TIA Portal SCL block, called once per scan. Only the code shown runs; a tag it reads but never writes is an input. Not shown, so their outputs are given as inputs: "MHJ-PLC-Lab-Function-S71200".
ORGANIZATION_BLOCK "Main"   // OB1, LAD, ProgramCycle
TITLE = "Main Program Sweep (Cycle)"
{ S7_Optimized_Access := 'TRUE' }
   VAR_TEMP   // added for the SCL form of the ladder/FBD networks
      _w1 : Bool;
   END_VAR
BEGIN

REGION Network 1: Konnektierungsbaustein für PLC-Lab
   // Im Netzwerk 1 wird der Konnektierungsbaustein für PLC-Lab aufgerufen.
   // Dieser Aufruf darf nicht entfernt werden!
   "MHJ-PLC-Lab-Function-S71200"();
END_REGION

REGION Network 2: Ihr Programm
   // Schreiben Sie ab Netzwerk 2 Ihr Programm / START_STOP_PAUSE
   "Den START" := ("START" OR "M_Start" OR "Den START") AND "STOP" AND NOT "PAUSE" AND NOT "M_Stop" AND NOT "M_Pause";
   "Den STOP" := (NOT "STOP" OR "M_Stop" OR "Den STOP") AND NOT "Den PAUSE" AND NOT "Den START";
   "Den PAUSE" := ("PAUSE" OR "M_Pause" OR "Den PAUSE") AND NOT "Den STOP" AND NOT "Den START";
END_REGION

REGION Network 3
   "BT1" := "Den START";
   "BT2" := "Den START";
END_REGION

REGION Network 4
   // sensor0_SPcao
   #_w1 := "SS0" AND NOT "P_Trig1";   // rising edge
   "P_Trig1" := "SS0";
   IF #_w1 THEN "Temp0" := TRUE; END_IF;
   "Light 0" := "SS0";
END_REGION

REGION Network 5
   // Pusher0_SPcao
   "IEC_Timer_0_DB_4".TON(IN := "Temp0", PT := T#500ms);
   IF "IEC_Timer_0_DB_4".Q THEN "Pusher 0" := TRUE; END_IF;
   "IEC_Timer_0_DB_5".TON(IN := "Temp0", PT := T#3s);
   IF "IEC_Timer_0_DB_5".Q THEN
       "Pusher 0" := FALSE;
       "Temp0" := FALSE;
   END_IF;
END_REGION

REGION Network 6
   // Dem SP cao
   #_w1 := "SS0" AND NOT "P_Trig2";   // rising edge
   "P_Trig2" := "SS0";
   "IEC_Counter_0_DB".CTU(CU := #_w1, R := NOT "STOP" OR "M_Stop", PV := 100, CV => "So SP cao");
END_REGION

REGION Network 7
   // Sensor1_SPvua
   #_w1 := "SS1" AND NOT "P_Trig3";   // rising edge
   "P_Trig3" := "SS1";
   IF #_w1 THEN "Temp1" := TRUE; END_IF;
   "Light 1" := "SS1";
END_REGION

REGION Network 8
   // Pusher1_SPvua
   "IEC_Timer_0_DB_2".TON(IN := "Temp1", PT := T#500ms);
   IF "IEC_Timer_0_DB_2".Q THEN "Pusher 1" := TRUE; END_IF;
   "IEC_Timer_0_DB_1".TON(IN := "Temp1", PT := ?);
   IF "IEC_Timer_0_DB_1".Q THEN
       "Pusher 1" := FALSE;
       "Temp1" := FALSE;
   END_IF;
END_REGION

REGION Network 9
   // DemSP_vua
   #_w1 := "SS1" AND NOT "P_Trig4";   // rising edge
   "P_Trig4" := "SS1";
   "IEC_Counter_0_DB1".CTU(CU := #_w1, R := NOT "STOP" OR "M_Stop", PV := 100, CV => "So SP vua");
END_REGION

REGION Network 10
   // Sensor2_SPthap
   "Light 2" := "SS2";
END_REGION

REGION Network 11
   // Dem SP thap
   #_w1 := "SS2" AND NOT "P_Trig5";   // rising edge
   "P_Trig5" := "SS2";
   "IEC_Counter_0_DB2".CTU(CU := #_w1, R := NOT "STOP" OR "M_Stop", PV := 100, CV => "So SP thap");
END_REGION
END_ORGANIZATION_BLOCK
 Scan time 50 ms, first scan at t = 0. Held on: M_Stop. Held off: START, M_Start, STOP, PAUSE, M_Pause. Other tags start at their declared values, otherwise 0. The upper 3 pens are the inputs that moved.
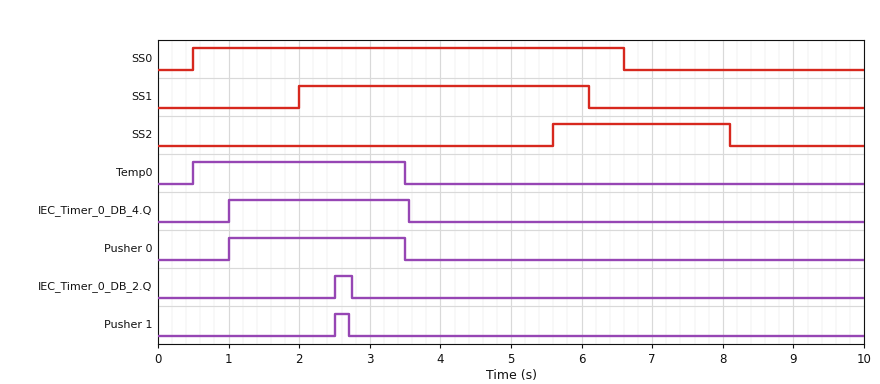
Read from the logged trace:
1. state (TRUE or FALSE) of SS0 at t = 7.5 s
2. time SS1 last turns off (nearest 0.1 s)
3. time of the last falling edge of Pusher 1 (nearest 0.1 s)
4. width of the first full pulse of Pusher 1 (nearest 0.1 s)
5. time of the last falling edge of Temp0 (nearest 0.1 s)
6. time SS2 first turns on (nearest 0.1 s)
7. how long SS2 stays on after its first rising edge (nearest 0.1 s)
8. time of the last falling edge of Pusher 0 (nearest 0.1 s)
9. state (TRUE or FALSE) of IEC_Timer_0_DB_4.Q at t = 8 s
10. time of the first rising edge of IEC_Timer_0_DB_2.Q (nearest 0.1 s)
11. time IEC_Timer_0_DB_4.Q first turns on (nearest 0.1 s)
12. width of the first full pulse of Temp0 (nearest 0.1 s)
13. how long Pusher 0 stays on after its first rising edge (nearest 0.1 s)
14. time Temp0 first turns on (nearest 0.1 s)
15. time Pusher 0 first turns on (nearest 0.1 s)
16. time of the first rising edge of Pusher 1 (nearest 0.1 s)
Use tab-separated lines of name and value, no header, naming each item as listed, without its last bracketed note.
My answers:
state (TRUE or FALSE) of SS0 at t = 7.5 s	FALSE
time SS1 last turns off	6.1 s
time of the last falling edge of Pusher 1	2.7 s
width of the first full pulse of Pusher 1	0.2 s
time of the last falling edge of Temp0	3.5 s
time SS2 first turns on	5.6 s
how long SS2 stays on after its first rising edge	2.5 s
time of the last falling edge of Pusher 0	3.5 s
state (TRUE or FALSE) of IEC_Timer_0_DB_4.Q at t = 8 s	FALSE
time of the first rising edge of IEC_Timer_0_DB_2.Q	2.5 s
time IEC_Timer_0_DB_4.Q first turns on	1.0 s
width of the first full pulse of Temp0	3.0 s
how long Pusher 0 stays on after its first rising edge	2.5 s
time Temp0 first turns on	0.5 s
time Pusher 0 first turns on	1.0 s
time of the first rising edge of Pusher 1	2.5 s
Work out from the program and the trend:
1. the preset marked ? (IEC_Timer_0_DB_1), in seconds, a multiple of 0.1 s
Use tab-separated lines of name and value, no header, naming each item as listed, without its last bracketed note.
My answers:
the preset marked ? (IEC_Timer_0_DB_1), in seconds, a multiple of 0.1 s	0.7 s
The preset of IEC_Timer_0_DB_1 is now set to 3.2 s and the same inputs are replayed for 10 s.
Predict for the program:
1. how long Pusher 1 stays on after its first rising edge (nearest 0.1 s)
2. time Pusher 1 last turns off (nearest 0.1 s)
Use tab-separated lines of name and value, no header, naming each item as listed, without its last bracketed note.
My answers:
how long Pusher 1 stays on after its first rising edge	2.7 s
time Pusher 1 last turns off	5.2 s
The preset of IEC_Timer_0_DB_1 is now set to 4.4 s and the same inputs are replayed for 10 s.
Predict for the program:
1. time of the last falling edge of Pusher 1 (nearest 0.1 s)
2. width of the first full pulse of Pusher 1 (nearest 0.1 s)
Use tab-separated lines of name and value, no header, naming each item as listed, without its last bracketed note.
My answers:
time of the last falling edge of Pusher 1	6.4 s
width of the first full pulse of Pusher 1	3.9 s
